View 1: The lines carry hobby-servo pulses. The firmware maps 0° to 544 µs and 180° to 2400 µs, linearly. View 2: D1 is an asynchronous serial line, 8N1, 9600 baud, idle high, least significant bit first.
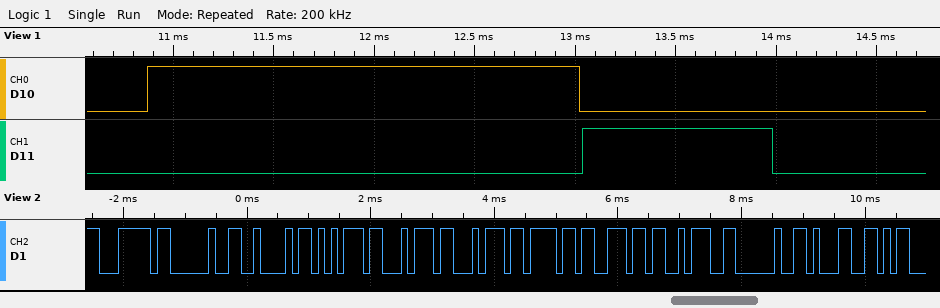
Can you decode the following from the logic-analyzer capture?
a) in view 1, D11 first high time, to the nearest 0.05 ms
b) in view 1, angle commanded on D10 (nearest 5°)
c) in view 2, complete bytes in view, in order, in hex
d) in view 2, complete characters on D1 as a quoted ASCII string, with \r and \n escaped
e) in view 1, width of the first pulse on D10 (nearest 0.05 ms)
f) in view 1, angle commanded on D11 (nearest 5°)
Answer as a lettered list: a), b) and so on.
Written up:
a) 0.95 ms
b) 155°
c) 7C 20 42 75 74 74 6F 6E 3A 20 31
d) "| Button: 1"
e) 2.15 ms
f) 40°
